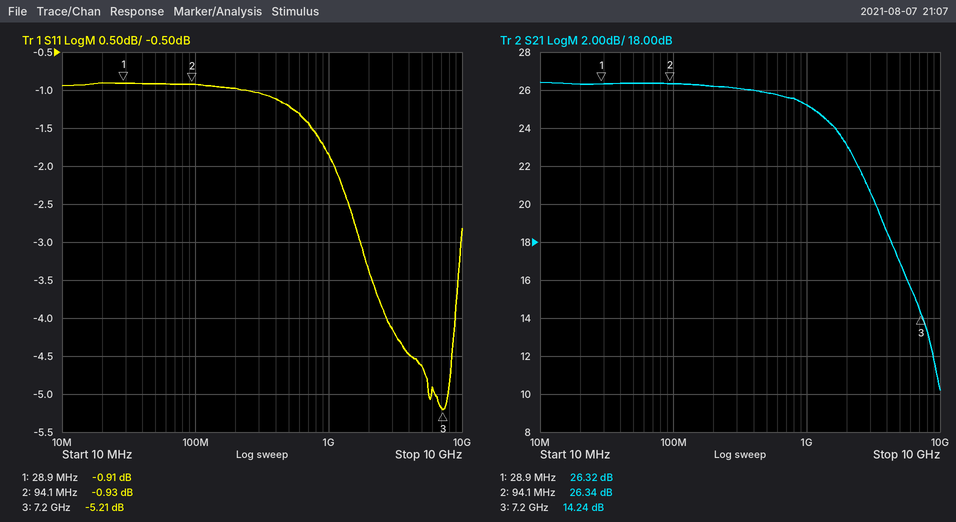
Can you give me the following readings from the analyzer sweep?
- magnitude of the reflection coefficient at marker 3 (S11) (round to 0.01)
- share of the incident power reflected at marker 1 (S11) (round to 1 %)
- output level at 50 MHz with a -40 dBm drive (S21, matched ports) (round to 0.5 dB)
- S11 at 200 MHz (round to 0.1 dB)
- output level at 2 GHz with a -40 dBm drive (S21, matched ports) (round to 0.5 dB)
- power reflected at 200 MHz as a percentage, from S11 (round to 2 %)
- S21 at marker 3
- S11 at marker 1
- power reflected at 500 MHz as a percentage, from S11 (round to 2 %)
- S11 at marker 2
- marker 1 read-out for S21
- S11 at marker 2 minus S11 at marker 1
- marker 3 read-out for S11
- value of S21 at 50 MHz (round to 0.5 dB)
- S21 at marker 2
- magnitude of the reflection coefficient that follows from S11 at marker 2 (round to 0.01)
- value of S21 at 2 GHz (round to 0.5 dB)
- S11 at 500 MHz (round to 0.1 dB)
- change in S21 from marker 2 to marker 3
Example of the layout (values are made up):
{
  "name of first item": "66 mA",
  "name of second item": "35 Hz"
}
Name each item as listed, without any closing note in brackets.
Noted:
{
  "magnitude of the reflection coefficient at marker 3 (S11)": "0.55",
  "share of the incident power reflected at marker 1 (S11)": "81 %",
  "output level at 50 MHz with a -40 dBm drive (S21, matched ports)": "-13.5 dBm",
  "S11 at 200 MHz": "-1.0 dB",
  "output level at 2 GHz with a -40 dBm drive (S21, matched ports)": "-17.0 dBm",
  "power reflected at 200 MHz as a percentage, from S11": "80 %",
  "S21 at marker 3": "14.24 dB",
  "S11 at marker 1": "-0.91 dB",
  "power reflected at 500 MHz as a percentage, from S11": "76 %",
  "S11 at marker 2": "-0.93 dB",
  "marker 1 read-out for S21": "26.32 dB",
  "S11 at marker 2 minus S11 at marker 1": "-0.02 dB",
  "marker 3 read-out for S11": "-5.21 dB",
  "value of S21 at 50 MHz": "26.5 dB",
  "S21 at marker 2": "26.34 dB",
  "magnitude of the reflection coefficient that follows from S11 at marker 2": "0.90",
  "value of S21 at 2 GHz": "23.0 dB",
  "S11 at 500 MHz": "-1.2 dB",
  "change in S21 from marker 2 to marker 3": "-12.10 dB"
}
